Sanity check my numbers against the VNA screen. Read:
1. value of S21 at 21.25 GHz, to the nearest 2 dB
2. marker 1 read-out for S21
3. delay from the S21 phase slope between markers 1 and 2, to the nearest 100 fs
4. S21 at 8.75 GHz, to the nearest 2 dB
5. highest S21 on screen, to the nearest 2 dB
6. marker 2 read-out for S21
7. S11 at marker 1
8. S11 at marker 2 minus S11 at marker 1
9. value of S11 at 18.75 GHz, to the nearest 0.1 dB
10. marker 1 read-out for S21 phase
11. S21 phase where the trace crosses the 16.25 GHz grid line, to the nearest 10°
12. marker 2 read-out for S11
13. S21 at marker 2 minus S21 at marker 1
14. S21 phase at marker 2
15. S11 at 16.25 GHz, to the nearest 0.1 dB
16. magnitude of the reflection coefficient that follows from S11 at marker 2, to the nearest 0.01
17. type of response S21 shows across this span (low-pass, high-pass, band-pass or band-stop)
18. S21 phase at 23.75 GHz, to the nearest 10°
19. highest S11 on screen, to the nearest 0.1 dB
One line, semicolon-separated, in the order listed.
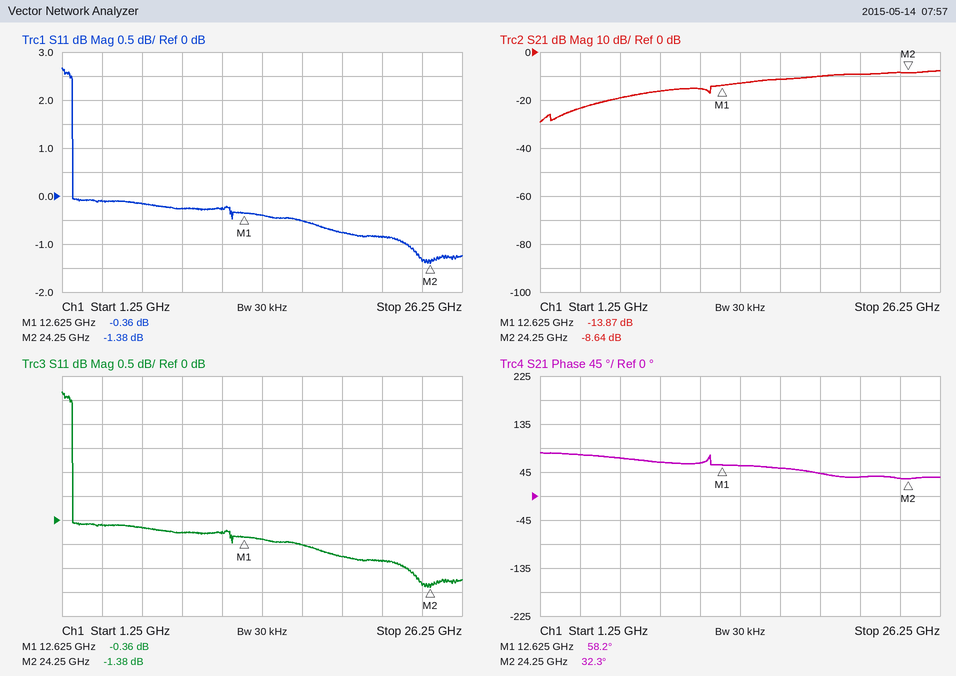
-10 dB; -13.87 dB; 6.2 ps; -16 dB; -8 dB; -8.64 dB; -0.36 dB; -1.02 dB; -0.8 dB; 58.2°; 50°; -1.38 dB; 5.23 dB; 32.3°; -0.5 dB; 0.85; high-pass; 30°; 2.7 dB
